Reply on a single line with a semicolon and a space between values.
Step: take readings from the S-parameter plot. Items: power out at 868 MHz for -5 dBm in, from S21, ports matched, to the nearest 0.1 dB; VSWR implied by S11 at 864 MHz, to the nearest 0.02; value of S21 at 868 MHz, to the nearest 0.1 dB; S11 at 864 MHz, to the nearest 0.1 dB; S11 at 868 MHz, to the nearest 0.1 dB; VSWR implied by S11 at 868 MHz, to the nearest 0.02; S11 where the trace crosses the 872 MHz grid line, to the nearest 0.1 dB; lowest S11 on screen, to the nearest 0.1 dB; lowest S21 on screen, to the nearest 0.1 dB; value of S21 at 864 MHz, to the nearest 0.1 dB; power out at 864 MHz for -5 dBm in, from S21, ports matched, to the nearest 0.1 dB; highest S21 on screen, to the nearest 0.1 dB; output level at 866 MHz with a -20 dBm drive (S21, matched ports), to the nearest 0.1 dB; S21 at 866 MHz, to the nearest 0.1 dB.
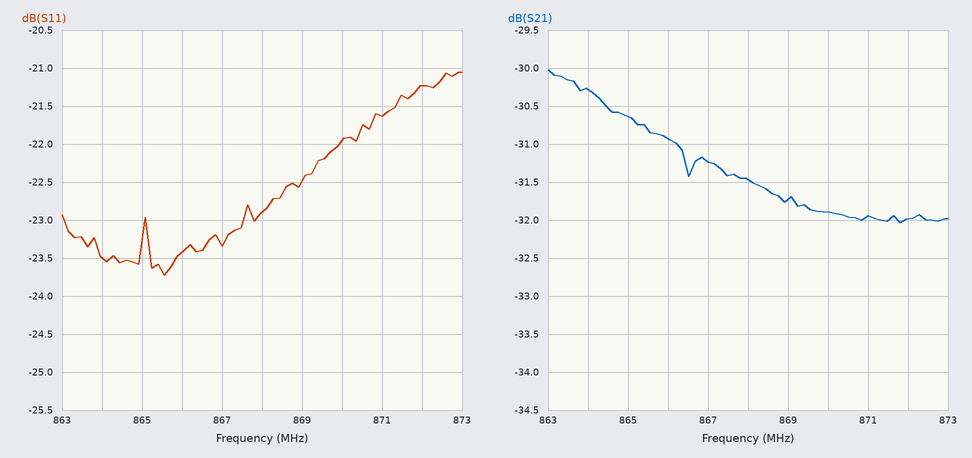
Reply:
-36.5 dBm; 1.14; -31.5 dB; -23.5 dB; -22.9 dB; 1.16; -21.2 dB; -23.7 dB; -32.0 dB; -30.3 dB; -35.3 dBm; -30.0 dB; -50.9 dBm; -30.9 dB
